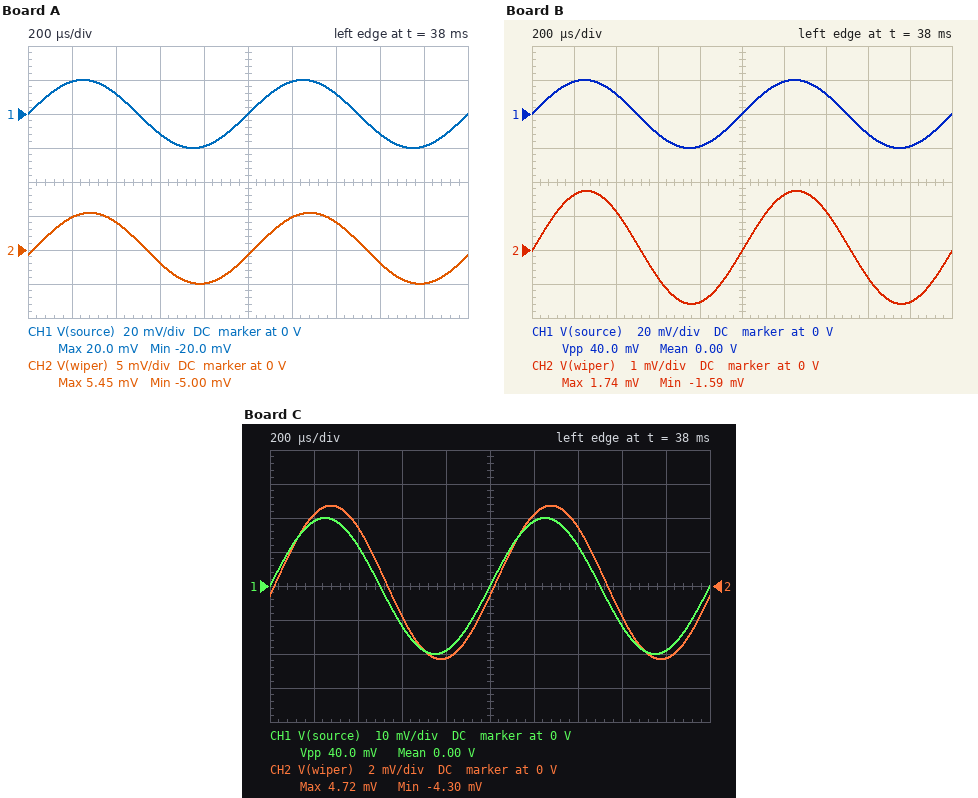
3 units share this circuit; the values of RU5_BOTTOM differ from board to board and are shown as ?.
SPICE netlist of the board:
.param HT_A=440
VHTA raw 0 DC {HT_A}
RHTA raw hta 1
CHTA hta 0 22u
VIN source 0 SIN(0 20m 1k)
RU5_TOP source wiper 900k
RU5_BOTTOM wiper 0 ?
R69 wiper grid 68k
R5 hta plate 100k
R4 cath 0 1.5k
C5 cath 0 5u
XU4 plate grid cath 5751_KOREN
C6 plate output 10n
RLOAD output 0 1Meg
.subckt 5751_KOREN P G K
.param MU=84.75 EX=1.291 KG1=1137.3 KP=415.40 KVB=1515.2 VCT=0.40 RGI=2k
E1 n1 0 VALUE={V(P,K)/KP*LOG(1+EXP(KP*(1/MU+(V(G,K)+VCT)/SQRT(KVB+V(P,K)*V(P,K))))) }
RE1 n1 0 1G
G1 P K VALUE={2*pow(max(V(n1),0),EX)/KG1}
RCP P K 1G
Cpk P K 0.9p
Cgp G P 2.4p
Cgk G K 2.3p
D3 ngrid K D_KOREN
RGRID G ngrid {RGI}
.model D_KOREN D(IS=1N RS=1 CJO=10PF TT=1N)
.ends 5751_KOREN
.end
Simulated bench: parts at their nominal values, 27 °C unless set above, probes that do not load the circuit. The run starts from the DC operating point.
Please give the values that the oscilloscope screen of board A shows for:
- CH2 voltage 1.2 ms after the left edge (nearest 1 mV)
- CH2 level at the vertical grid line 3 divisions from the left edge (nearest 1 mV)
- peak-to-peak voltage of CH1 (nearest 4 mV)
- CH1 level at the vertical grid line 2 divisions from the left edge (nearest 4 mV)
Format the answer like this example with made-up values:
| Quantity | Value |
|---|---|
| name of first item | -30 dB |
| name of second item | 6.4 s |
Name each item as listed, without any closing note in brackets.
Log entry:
| Quantity | Value |
|---|---|
| CH2 voltage 1.2 ms after the left edge | 5 mV |
| CH2 level at the vertical grid line 3 divisions from the left edge | -2 mV |
| peak-to-peak voltage of CH1 | 40 mV |
| CH1 level at the vertical grid line 2 divisions from the left edge | 12 mV |
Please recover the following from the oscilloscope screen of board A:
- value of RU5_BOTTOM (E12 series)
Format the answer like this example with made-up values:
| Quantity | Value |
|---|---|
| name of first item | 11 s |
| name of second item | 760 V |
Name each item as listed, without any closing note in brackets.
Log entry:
| Quantity | Value |
|---|---|
| value of RU5_BOTTOM | 330 kΩ |
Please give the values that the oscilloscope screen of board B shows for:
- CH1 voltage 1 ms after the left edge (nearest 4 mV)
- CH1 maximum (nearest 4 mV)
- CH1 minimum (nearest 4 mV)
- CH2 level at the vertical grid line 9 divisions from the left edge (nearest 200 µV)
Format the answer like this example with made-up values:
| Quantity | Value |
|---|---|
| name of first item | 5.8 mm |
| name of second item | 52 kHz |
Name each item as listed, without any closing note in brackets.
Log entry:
| Quantity | Value |
|---|---|
| CH1 voltage 1 ms after the left edge | 0 V |
| CH1 maximum | 20 mV |
| CH1 minimum | -20 mV |
| CH2 level at the vertical grid line 9 divisions from the left edge | -1.6 mV |
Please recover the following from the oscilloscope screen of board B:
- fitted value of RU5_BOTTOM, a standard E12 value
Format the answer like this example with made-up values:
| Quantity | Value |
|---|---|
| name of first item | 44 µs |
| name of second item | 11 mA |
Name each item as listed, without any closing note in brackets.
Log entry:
| Quantity | Value |
|---|---|
| fitted value of RU5_BOTTOM, a standard E12 value | 82 kΩ |
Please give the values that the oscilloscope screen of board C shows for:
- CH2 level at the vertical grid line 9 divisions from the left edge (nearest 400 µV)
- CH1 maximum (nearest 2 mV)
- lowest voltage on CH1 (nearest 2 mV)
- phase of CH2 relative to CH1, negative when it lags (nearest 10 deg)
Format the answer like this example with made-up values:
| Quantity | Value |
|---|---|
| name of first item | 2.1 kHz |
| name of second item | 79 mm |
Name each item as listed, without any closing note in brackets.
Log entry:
| Quantity | Value |
|---|---|
| CH2 level at the vertical grid line 9 divisions from the left edge | -4.4 mV |
| CH1 maximum | 20 mV |
| lowest voltage on CH1 | -20 mV |
| phase of CH2 relative to CH1, negative when it lags | -10 deg |
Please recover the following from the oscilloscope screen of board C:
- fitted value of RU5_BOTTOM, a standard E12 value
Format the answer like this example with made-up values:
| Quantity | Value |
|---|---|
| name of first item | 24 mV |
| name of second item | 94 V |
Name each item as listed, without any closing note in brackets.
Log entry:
| Quantity | Value |
|---|---|
| fitted value of RU5_BOTTOM, a standard E12 value | 270 kΩ |
